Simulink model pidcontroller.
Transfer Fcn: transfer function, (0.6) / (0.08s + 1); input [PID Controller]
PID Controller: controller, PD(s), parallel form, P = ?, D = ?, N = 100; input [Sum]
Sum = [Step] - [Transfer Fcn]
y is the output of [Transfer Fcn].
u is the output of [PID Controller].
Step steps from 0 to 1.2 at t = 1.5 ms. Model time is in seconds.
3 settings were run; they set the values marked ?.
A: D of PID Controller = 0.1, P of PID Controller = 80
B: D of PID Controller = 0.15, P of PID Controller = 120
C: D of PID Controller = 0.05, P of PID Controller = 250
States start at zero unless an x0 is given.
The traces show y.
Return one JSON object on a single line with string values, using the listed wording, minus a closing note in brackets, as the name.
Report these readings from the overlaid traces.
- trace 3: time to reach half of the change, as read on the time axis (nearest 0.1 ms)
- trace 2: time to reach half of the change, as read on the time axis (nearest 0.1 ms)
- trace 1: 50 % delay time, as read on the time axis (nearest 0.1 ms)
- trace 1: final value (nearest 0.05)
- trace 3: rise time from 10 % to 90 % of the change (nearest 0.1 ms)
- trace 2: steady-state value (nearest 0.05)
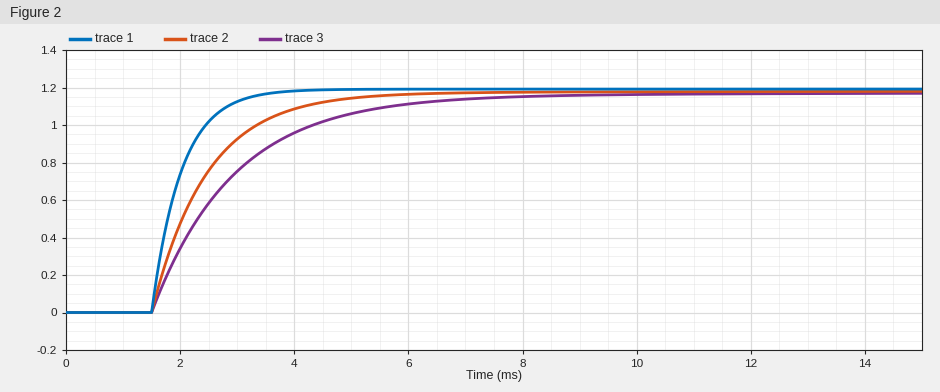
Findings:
{"trace 3: time to reach half of the change, as read on the time axis": "2.5 ms", "trace 2: time to reach half of the change, as read on the time axis": "2.2 ms", "trace 1: 50 % delay time, as read on the time axis": "1.9 ms", "trace 1: final value": "1.20", "trace 3: rise time from 10 % to 90 % of the change": "3.3 ms", "trace 2: steady-state value": "1.20"}
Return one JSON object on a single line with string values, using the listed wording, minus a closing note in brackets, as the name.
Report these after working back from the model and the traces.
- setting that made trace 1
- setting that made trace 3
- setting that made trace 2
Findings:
{"setting that made trace 1": "C", "setting that made trace 3": "A", "setting that made trace 2": "B"}
